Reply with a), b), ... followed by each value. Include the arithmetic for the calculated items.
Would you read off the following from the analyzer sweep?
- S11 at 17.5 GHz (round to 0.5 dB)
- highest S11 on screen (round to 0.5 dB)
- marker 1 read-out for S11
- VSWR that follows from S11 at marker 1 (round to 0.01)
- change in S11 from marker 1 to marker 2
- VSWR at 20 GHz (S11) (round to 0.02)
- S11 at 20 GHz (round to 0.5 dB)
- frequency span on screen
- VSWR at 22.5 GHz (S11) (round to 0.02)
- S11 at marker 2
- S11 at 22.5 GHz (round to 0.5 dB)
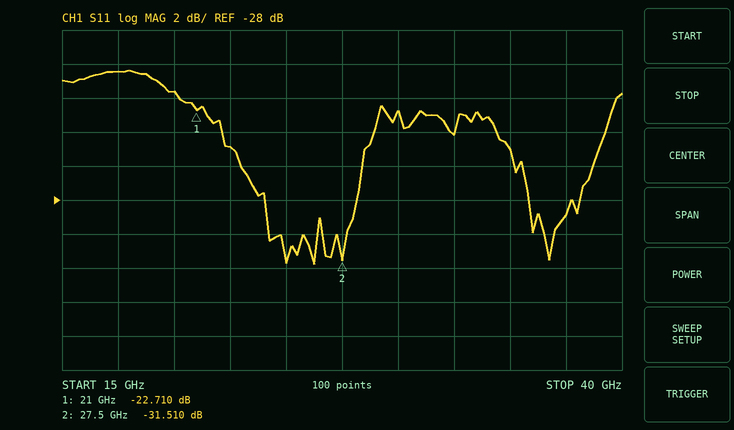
a) -20.5 dB
b) -20.5 dB
c) -22.710 dB
d) (1 + 0.0732)/(1 − 0.0732) ≈ 1.16
e) -31.51 − (-22.71) = -8.800 dB
f) |Γ| = 10^(-21.5/20) = 0.0841; VSWR = (1 + 0.0841)/(1 − 0.0841) ≈ 1.18
g) -21.5 dB
h) 25 GHz
i) |Γ| = 10^(-25/20) = 0.0562; VSWR = (1 + 0.0562)/(1 − 0.0562) ≈ 1.12
j) -31.510 dB
k) -25.0 dB
